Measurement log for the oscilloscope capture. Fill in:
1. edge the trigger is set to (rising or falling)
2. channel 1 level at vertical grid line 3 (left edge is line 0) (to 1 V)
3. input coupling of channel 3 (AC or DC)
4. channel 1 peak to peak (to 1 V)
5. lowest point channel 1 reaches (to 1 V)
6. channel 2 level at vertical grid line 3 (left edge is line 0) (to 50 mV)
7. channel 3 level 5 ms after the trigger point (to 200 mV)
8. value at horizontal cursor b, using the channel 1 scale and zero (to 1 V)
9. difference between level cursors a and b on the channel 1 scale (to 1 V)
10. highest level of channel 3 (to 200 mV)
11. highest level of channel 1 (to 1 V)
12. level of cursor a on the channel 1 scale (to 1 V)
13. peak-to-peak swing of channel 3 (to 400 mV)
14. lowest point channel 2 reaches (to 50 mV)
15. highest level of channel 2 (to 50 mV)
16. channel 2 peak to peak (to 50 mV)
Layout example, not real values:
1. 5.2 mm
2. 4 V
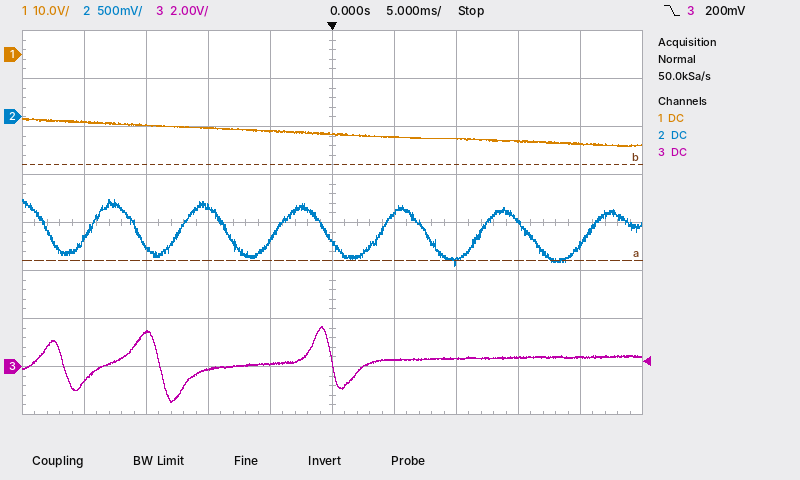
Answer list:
1. falling
2. -15 V
3. DC
4. 6 V
5. -19 V
6. -950 mV
7. 200 mV
8. -23 V
9. 20 V
10. 1.6 V
11. -13 V
12. -43 V
13. 3.2 V
14. -1.55 V
15. -850 mV
16. 700 mV
